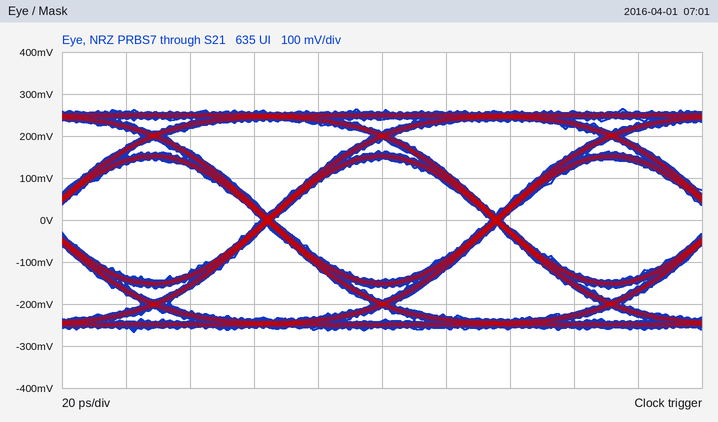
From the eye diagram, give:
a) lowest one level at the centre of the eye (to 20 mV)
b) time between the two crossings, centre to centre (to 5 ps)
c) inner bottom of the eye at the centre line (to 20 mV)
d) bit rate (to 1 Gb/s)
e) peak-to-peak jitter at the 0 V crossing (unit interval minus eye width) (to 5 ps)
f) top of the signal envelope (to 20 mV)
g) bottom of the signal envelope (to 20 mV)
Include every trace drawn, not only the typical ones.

140 mV
70 ps
-140 mV
14 Gb/s
5 ps
260 mV
-260 mV
